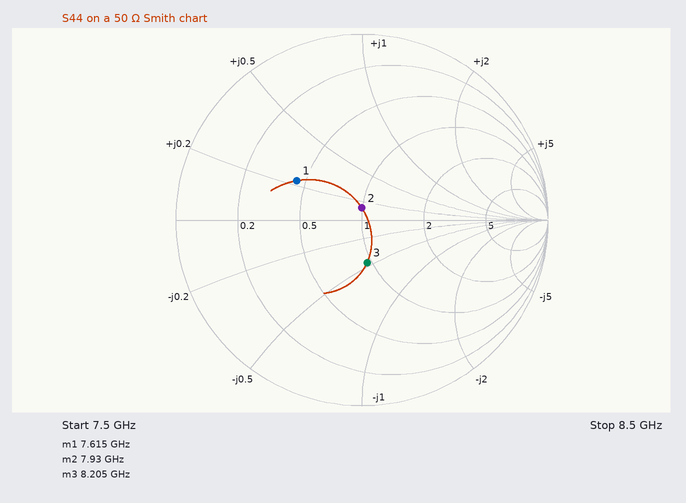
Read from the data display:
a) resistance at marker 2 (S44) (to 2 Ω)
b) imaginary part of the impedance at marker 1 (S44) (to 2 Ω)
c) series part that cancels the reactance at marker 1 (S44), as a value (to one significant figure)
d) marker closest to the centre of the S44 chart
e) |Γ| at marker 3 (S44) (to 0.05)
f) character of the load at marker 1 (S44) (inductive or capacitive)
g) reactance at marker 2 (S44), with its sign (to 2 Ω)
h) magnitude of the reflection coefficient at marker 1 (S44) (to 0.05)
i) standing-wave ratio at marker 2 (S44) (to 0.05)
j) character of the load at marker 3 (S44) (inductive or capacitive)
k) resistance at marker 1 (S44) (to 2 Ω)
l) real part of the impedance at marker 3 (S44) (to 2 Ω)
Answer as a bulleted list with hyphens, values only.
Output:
- 50 Ω
- +12 Ω
- 2 pF
- marker 2
- 0.25
- inductive
- +6 Ω
- 0.40
- 1.15
- capacitive
- 22 Ω
- 48 Ω
